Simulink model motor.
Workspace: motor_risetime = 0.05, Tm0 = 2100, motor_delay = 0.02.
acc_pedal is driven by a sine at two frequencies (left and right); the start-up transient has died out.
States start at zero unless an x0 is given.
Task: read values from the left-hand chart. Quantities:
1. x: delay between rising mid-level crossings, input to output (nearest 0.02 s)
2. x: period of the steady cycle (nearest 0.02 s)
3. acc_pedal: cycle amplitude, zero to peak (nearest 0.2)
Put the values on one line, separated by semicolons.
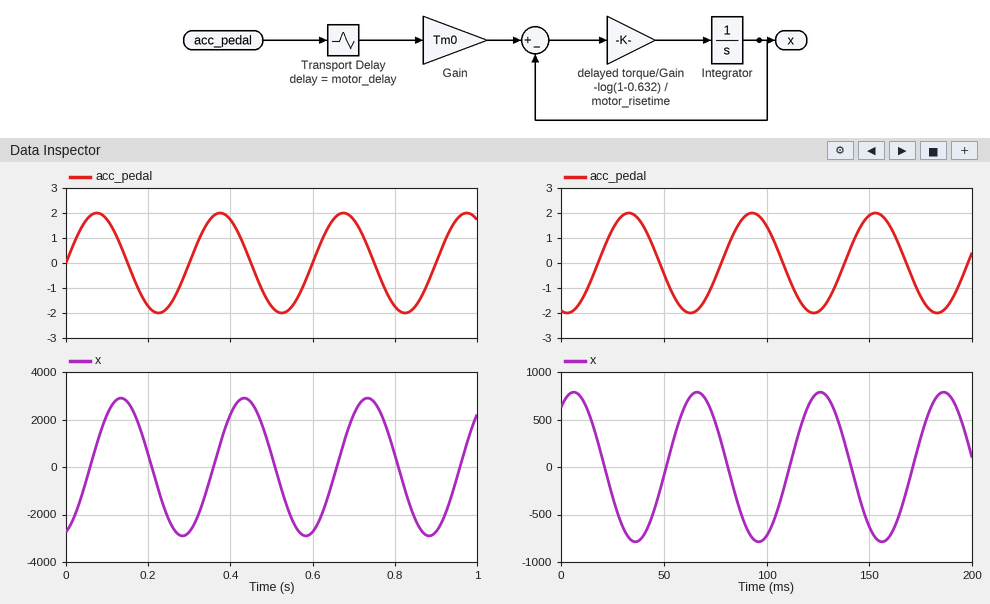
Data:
0.06 s; 0.30 s; 2.0
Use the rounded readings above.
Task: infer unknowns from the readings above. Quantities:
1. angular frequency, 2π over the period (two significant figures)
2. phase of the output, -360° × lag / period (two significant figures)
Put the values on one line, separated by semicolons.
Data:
21 rad/s; -72°
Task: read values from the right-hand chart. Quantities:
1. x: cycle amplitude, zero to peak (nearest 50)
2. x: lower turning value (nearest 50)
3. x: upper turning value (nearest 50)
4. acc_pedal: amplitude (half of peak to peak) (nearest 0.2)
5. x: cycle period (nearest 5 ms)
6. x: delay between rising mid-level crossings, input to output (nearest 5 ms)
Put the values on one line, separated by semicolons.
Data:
800; -800; 800; 2.0; 60 ms; 35 ms
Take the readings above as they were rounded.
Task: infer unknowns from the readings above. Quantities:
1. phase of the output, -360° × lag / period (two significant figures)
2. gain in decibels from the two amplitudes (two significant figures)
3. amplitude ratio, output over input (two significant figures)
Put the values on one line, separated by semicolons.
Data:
-210°; 52 dB; 400
